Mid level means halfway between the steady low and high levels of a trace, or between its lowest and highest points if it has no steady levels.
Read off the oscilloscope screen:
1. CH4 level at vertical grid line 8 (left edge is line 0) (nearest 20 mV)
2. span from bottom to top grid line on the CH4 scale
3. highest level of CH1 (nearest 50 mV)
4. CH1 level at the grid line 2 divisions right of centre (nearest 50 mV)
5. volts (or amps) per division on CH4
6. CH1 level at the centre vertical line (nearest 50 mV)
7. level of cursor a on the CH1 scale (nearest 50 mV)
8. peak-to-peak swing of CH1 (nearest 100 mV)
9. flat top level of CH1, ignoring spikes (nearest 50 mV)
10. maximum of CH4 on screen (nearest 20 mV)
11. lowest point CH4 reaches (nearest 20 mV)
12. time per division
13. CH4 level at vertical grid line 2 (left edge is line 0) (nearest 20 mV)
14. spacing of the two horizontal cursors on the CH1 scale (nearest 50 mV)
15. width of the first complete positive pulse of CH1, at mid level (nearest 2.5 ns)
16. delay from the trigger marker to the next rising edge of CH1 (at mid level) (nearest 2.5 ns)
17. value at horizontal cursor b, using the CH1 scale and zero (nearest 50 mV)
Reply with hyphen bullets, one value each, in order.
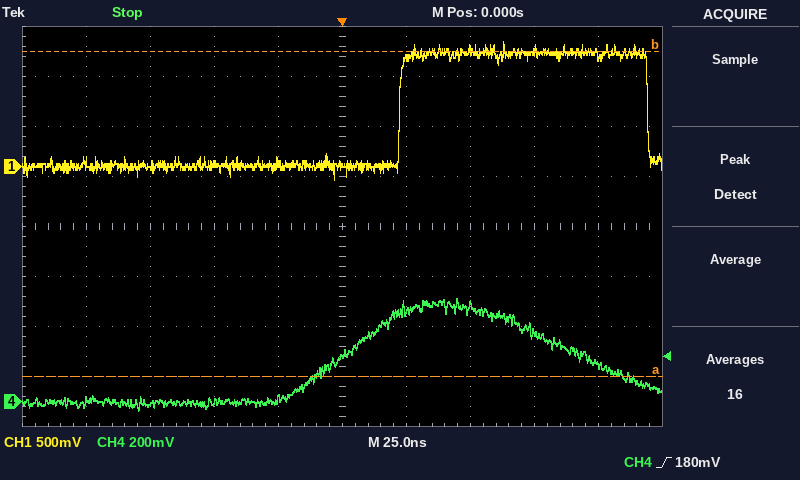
- 280 mV
- 1.6 V
- 1.25 V
- 1.15 V
- 200 mV
- 0 mV
- -2.10 V
- 1.40 V
- 1.15 V
- 420 mV
- -40 mV
- 25 ns
- 0 mV
- 3.25 V
- 97.5 ns
- 22.5 ns
- 1.15 V
